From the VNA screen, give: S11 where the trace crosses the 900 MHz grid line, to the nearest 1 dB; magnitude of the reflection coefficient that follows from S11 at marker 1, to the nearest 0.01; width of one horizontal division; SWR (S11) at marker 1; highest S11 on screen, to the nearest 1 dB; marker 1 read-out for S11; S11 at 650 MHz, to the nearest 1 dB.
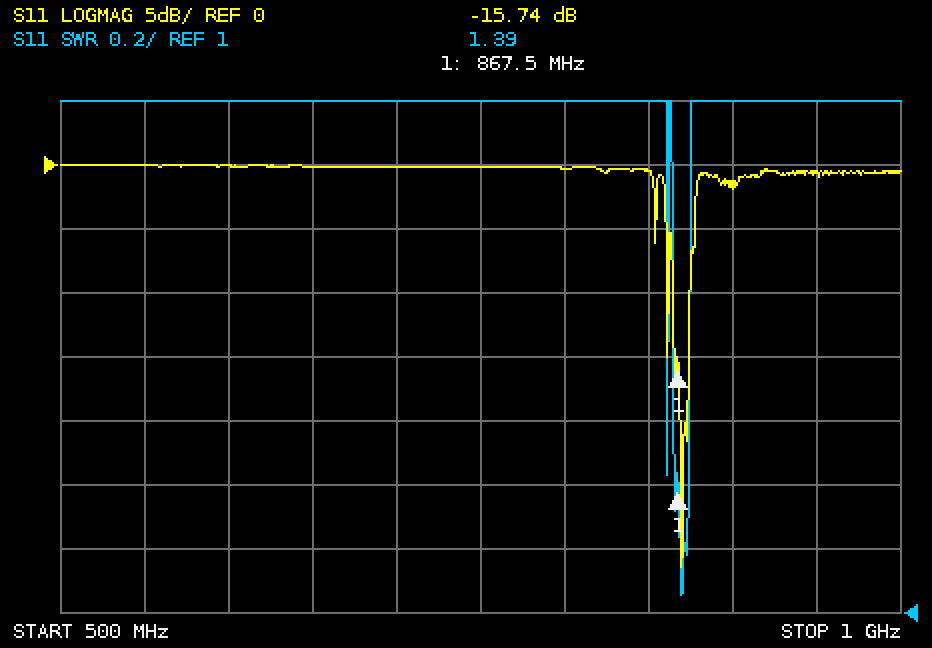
-2 dB
0.16
50 MHz
1.39
0 dB
-15.74 dB
0 dB
